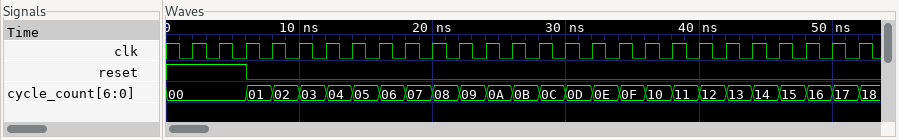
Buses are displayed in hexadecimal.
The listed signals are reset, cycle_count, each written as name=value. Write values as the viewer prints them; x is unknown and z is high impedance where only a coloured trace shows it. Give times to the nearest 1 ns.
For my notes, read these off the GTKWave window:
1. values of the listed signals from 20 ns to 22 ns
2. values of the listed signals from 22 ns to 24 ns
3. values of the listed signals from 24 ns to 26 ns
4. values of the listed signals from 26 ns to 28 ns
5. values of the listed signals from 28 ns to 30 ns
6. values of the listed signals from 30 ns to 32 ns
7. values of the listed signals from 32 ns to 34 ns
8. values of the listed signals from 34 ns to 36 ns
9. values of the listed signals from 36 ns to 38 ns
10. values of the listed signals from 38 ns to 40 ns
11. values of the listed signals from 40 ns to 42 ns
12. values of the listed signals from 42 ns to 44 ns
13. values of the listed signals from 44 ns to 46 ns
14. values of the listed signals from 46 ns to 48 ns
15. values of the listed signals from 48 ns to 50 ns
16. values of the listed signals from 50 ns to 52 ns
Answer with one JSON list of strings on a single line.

["reset=0, cycle_count=08", "reset=0, cycle_count=09", "reset=0, cycle_count=0A", "reset=0, cycle_count=0B", "reset=0, cycle_count=0C", "reset=0, cycle_count=0D", "reset=0, cycle_count=0E", "reset=0, cycle_count=0F", "reset=0, cycle_count=10", "reset=0, cycle_count=11", "reset=0, cycle_count=12", "reset=0, cycle_count=13", "reset=0, cycle_count=14", "reset=0, cycle_count=15", "reset=0, cycle_count=16", "reset=0, cycle_count=17"]
